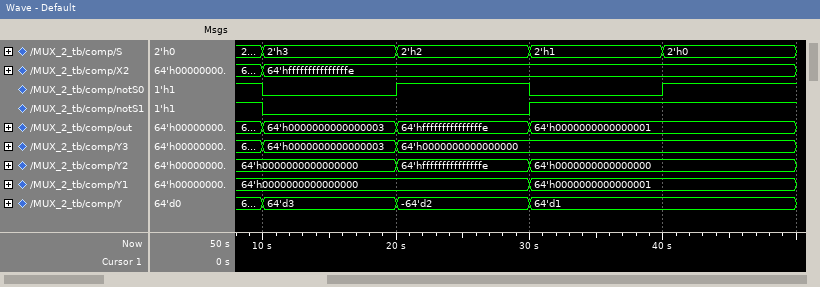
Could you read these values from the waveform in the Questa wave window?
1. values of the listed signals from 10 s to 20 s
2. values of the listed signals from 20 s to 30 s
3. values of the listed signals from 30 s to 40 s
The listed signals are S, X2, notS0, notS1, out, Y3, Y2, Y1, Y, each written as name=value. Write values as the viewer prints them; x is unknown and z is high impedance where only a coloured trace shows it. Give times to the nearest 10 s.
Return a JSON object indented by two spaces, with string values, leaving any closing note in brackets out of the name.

{
  "values of the listed signals from 10 s to 20 s": "S=2'h3, X2=64'hfffffffffffffffe, notS0=0, notS1=0, out=64'h0000000000000003, Y3=64'h0000000000000003, Y2=64'h0000000000000000, Y1=64'h0000000000000000, Y=64'd3",
  "values of the listed signals from 20 s to 30 s": "S=2'h2, X2=64'hfffffffffffffffe, notS0=1, notS1=0, out=64'hfffffffffffffffe, Y3=64'h0000000000000000, Y2=64'hfffffffffffffffe, Y1=64'h0000000000000000, Y=-64'd2",
  "values of the listed signals from 30 s to 40 s": "S=2'h1, X2=64'hfffffffffffffffe, notS0=0, notS1=1, out=64'h0000000000000001, Y3=64'h0000000000000000, Y2=64'h0000000000000000, Y1=64'h0000000000000001, Y=64'd1"
}
